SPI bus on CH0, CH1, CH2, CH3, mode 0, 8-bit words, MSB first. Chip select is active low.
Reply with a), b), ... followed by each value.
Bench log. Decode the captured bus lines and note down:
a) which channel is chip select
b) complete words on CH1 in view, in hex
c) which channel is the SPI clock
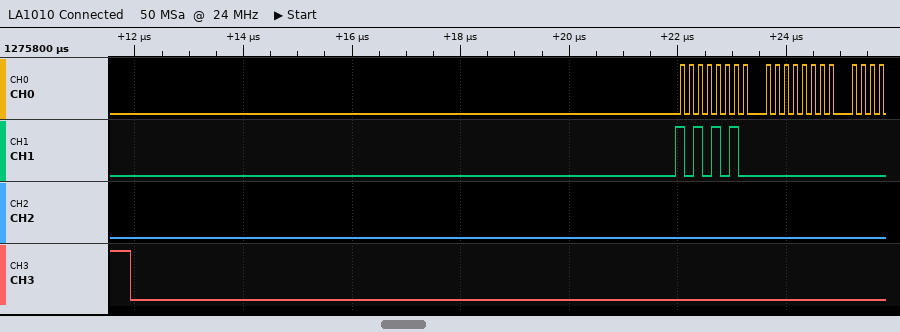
a) CH3
b) AA, 00
c) CH0
